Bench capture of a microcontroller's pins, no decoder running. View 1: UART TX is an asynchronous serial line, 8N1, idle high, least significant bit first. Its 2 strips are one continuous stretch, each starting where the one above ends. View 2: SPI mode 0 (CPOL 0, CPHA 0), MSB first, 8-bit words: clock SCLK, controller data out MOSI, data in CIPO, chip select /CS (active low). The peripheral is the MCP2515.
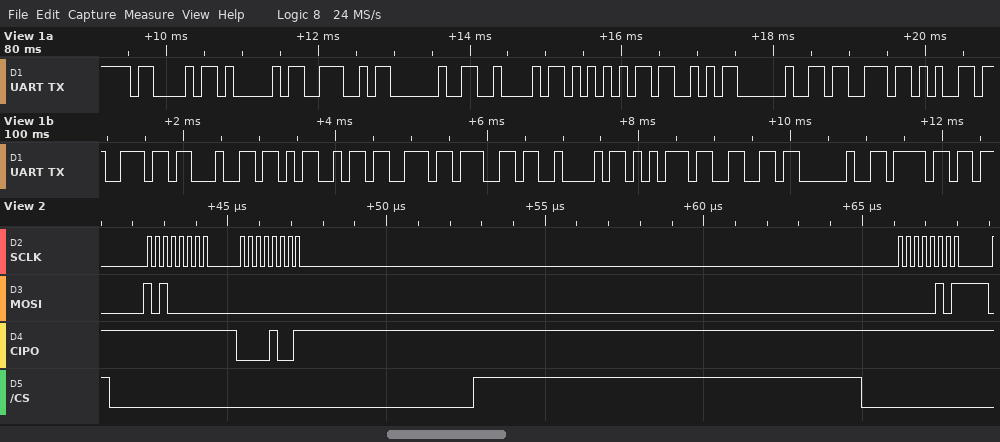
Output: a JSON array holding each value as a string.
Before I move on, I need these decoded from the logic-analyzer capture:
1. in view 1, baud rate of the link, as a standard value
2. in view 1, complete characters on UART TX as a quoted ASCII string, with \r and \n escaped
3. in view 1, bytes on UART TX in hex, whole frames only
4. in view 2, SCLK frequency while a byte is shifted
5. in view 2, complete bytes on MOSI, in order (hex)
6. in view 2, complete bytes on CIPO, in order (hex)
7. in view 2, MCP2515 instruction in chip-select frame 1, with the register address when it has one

["9600 baud", "\"CAN BUS sendMsgBuf o\"", "43 41 4E 20 42 55 53 20 73 65 6E 64 4D 73 67 42 75 66 20 6F", "4 MHz", "A0 00 05", "FF 09 FF", "READ STATUS"]
